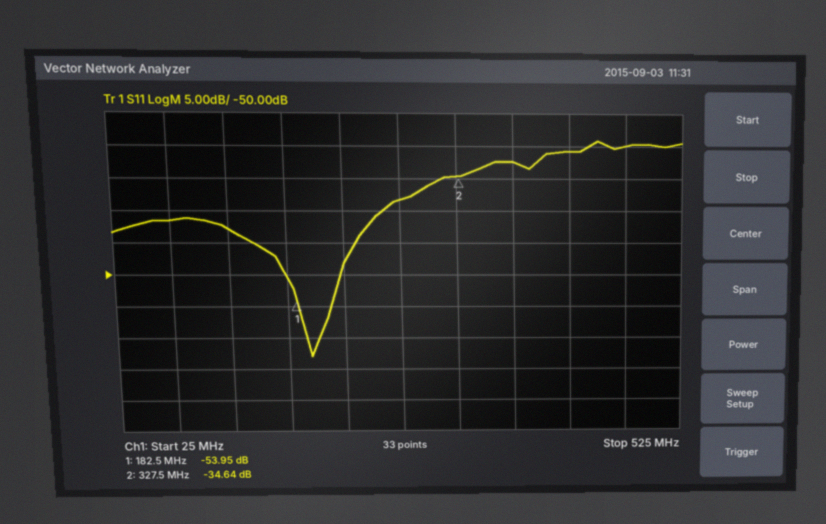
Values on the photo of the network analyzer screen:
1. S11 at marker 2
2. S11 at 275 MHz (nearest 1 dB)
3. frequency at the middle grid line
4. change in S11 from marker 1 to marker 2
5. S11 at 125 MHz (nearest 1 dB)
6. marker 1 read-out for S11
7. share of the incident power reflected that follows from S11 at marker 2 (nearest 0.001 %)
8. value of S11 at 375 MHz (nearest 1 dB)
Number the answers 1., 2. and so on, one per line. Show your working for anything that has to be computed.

1. -34.64 dB
2. -38 dB
3. 275 MHz
4. -34.64 − (-53.95) = 19.31 dB
5. -43 dB
6. -53.95 dB
7. 10^(-34.64/10) ≈ 0.034 %
8. -32 dB
